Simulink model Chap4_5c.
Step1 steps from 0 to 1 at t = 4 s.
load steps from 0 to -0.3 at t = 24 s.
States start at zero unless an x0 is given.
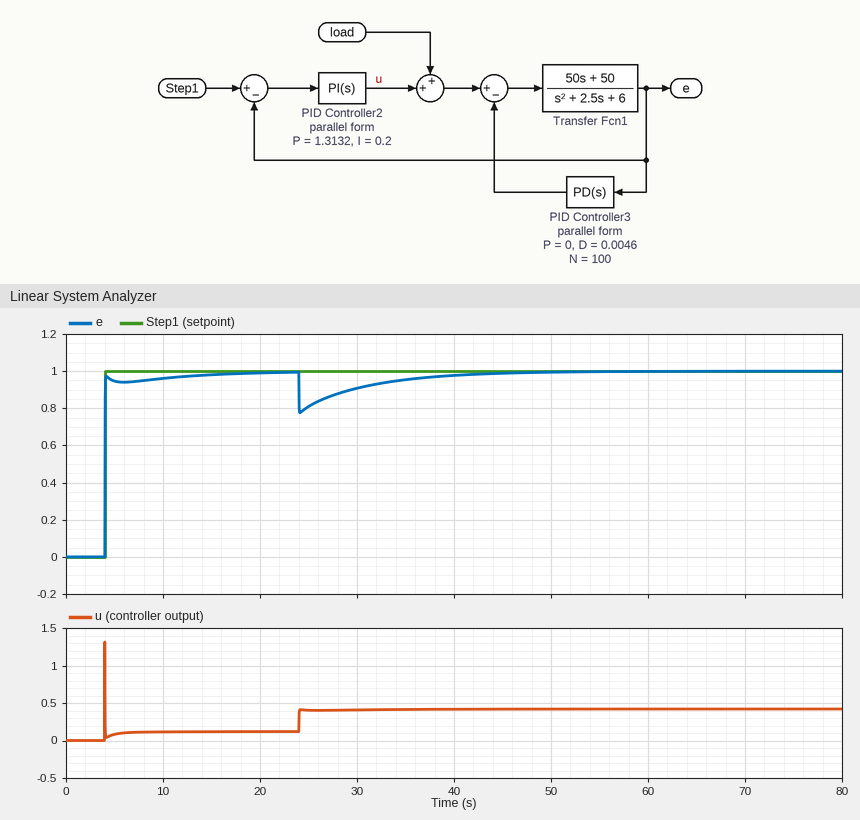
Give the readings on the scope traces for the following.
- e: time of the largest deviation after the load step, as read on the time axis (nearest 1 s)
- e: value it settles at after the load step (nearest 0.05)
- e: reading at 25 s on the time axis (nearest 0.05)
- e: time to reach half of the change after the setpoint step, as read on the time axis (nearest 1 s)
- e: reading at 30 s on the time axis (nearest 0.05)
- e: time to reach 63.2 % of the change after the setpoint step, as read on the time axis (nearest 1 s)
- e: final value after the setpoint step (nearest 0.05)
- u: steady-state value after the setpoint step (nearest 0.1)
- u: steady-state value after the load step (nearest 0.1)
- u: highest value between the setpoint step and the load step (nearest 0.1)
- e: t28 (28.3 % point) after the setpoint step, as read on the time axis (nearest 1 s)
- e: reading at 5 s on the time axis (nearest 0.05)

24 s
1.00
0.80
4 s
0.90
4 s
1.00
0.1
0.4
1.3
4 s
0.95
